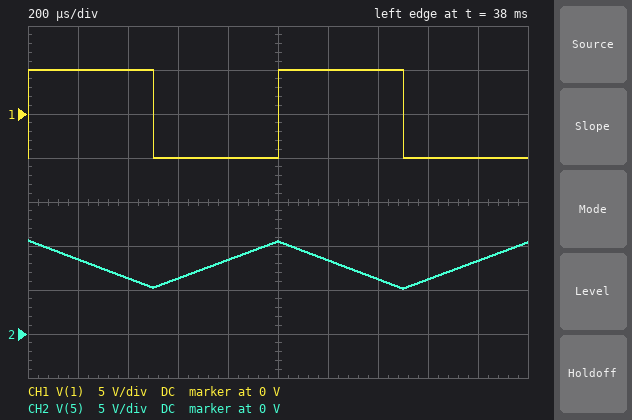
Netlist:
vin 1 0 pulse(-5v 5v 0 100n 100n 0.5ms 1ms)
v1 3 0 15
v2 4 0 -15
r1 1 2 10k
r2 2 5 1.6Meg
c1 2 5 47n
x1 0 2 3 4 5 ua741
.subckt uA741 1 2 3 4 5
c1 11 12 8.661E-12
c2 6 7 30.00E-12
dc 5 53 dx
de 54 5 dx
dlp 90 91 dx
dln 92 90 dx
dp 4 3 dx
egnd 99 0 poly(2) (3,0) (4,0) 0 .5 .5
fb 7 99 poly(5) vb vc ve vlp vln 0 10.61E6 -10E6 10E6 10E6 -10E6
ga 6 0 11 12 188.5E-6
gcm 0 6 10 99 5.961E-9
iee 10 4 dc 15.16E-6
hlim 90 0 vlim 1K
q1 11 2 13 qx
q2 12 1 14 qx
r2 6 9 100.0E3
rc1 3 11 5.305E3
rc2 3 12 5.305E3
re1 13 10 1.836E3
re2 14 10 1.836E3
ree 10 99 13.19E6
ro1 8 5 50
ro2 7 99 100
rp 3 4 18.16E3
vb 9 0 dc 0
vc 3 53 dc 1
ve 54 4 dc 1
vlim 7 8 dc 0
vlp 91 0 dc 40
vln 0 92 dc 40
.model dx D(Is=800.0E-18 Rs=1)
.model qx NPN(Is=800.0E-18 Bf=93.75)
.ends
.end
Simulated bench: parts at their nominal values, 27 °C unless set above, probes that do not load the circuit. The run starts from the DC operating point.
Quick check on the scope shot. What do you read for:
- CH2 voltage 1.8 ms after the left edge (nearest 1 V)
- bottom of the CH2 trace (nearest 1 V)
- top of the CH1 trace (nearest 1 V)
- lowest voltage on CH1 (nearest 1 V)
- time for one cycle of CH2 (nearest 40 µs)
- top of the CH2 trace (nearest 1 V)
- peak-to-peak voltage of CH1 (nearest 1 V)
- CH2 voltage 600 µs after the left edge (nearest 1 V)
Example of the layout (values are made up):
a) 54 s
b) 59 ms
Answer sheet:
a) 8 V
b) 5 V
c) 5 V
d) -5 V
e) 1.00 ms
f) 11 V
g) 10 V
h) 6 V
